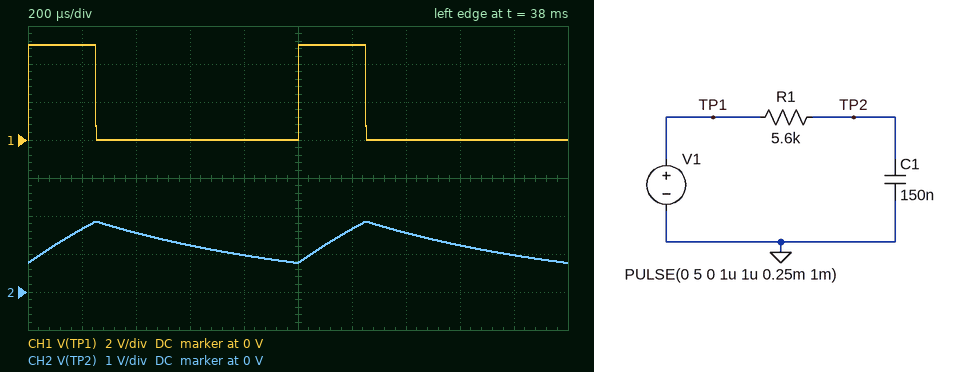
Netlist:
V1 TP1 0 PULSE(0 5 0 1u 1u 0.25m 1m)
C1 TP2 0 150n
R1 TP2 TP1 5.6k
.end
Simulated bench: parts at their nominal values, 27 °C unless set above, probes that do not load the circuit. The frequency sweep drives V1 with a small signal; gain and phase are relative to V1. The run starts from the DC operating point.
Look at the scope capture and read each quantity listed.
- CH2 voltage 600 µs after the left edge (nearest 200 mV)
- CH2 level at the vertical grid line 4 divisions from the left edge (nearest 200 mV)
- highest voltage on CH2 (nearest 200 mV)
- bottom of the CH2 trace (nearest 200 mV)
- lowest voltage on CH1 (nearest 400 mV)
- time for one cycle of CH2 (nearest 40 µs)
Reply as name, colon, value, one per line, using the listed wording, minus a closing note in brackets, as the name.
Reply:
CH2 voltage 600 µs after the left edge: 1.2 V
CH2 level at the vertical grid line 4 divisions from the left edge: 1.0 V
highest voltage on CH2: 1.8 V
bottom of the CH2 trace: 800 mV
lowest voltage on CH1: 0 V
time for one cycle of CH2: 1.00 ms
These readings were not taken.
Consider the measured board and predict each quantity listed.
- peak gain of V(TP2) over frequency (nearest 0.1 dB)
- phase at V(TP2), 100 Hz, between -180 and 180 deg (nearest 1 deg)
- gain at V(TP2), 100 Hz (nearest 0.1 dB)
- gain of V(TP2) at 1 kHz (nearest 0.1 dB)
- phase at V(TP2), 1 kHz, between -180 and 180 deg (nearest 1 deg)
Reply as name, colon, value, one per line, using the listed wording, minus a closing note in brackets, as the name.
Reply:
peak gain of V(TP2) over frequency: 0 dB
phase at V(TP2), 100 Hz, between -180 and 180 deg: -28 deg
gain at V(TP2), 100 Hz: -1.1 dB
gain of V(TP2) at 1 kHz: -14.6 dB
phase at V(TP2), 1 kHz, between -180 and 180 deg: -79 deg
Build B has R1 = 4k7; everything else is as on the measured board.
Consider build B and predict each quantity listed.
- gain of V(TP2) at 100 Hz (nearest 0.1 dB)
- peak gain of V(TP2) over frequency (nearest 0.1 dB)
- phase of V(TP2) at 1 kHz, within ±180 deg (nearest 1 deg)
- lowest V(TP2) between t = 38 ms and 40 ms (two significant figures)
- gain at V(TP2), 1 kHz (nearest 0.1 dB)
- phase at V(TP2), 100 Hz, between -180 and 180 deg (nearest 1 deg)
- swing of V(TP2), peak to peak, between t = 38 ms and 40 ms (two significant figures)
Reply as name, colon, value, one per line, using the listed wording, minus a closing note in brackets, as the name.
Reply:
gain of V(TP2) at 100 Hz: -0.8 dB
peak gain of V(TP2) over frequency: 0 dB
phase of V(TP2) at 1 kHz, within ±180 deg: -77 deg
lowest V(TP2) between t = 38 ms and 40 ms: 680 mV
gain at V(TP2), 1 kHz: -13.1 dB
phase at V(TP2), 100 Hz, between -180 and 180 deg: -24 deg
swing of V(TP2), peak to peak, between t = 38 ms and 40 ms: 1.3 V
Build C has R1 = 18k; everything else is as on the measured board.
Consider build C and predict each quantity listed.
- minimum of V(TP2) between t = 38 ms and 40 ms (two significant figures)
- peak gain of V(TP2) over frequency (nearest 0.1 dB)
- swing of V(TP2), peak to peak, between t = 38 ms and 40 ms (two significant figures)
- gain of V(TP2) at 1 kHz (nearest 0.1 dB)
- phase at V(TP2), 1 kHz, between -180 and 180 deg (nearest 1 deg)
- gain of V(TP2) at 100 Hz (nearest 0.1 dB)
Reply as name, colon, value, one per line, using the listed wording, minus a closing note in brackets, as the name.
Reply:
minimum of V(TP2) between t = 38 ms and 40 ms: 1.1 V
peak gain of V(TP2) over frequency: 0 dB
swing of V(TP2), peak to peak, between t = 38 ms and 40 ms: 350 mV
gain of V(TP2) at 1 kHz: -24.6 dB
phase at V(TP2), 1 kHz, between -180 and 180 deg: -87 deg
gain of V(TP2) at 100 Hz: -5.9 dB
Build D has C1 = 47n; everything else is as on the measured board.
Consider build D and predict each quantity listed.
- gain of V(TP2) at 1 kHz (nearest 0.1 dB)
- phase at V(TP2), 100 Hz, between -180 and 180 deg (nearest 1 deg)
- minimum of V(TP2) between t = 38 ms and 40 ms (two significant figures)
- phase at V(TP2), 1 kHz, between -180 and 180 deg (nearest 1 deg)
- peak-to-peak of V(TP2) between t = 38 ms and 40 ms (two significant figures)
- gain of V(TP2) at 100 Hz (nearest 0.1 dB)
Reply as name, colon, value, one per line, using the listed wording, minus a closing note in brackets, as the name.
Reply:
gain of V(TP2) at 1 kHz: -5.7 dB
phase at V(TP2), 100 Hz, between -180 and 180 deg: -9 deg
minimum of V(TP2) between t = 38 ms and 40 ms: 180 mV
phase at V(TP2), 1 kHz, between -180 and 180 deg: -59 deg
peak-to-peak of V(TP2) between t = 38 ms and 40 ms: 3.0 V
gain of V(TP2) at 100 Hz: -0.1 dB
